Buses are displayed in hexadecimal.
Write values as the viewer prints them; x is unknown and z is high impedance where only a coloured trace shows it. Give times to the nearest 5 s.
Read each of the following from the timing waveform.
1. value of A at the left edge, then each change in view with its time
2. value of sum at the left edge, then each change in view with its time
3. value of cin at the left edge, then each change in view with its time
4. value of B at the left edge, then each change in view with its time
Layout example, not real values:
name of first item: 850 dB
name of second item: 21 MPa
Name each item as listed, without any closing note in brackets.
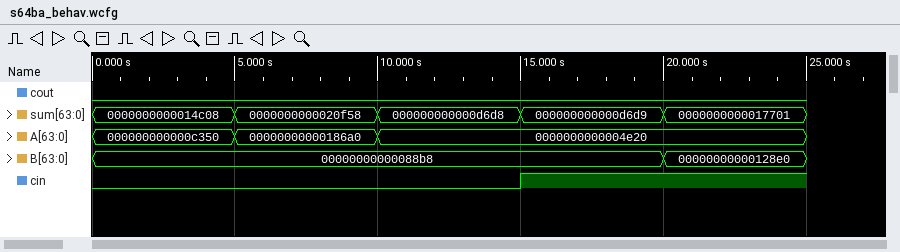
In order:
value of A at the left edge, then each change in view with its time: 000000000000c350, 00000000000186a0 at 5 s, 0000000000004e20 at 10 s
value of sum at the left edge, then each change in view with its time: 0000000000014c08, 0000000000020f58 at 5 s, 000000000000d6d8 at 10 s, 000000000000d6d9 at 15 s, 0000000000017701 at 20 s
value of cin at the left edge, then each change in view with its time: 0, 1 at 15 s
value of B at the left edge, then each change in view with its time: 00000000000088b8, 00000000000128e0 at 20 s
